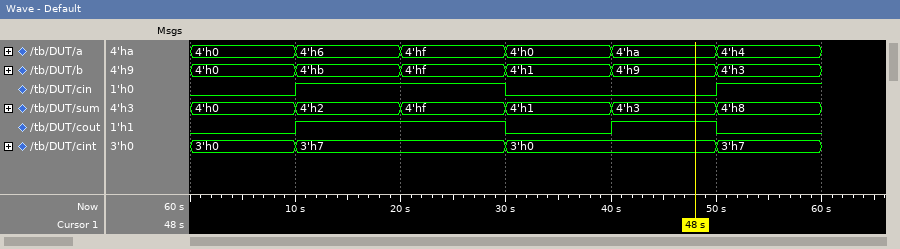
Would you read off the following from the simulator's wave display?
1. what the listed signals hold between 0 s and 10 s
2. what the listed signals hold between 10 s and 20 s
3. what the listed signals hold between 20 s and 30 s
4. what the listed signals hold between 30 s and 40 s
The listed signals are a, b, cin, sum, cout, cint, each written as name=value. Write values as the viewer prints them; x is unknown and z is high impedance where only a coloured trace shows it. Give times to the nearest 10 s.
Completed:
a=4'h0, b=4'h0, cin=0, sum=4'h0, cout=0, cint=3'h0
a=4'h6, b=4'hb, cin=1, sum=4'h2, cout=1, cint=3'h7
a=4'hf, b=4'hf, cin=1, sum=4'hf, cout=1, cint=3'h7
a=4'h0, b=4'h1, cin=0, sum=4'h1, cout=0, cint=3'h0
